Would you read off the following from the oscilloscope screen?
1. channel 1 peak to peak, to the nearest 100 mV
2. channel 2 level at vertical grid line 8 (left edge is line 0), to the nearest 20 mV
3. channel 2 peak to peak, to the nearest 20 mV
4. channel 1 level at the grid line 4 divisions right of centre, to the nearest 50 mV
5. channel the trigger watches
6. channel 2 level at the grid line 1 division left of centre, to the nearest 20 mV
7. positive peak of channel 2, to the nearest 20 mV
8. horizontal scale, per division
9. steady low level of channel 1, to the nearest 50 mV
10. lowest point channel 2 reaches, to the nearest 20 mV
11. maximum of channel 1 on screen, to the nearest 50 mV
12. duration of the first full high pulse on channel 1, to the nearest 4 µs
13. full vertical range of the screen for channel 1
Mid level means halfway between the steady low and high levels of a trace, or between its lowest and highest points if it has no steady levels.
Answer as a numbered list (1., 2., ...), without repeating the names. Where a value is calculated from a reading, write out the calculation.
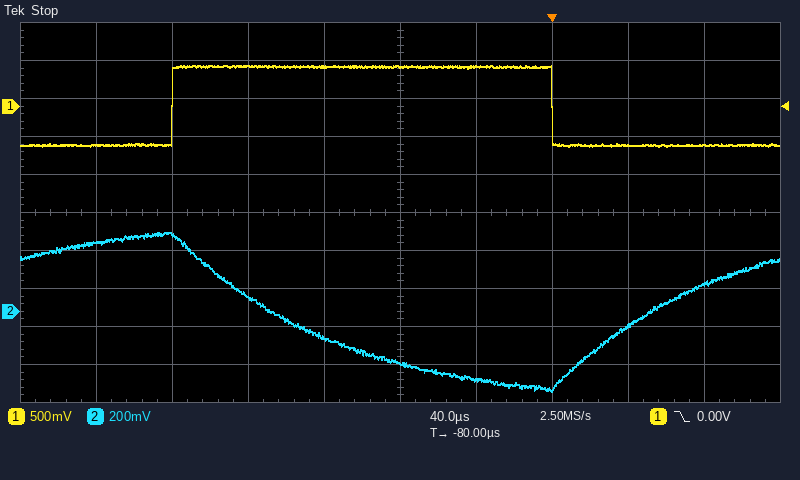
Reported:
1. 1.10 V
2. -80 mV
3. 420 mV − (-420 mV) = 840 mV
4. -500 mV
5. channel 1
6. -140 mV
7. 420 mV
8. 40 µs
9. -500 mV
10. -420 mV
11. 550 mV
12. 200 µs
13. 5 V
